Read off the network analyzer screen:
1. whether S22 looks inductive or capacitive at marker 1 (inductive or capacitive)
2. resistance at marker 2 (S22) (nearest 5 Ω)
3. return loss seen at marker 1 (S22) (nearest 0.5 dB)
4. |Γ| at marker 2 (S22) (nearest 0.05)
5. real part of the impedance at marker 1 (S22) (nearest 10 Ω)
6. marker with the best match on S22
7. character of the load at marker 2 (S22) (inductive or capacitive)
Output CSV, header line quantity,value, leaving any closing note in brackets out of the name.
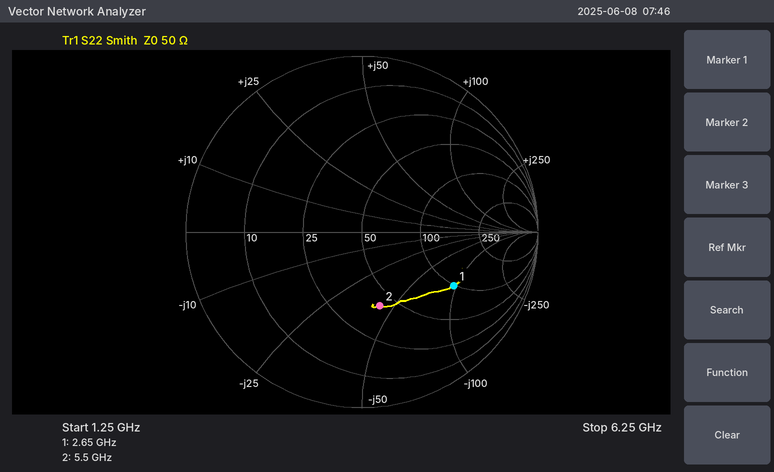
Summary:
quantity,value
whether S22 looks inductive or capacitive at marker 1,capacitive
resistance at marker 2 (S22),40 Ω
return loss seen at marker 1 (S22),4.5 dB
|Γ| at marker 2 (S22),0.45
real part of the impedance at marker 1 (S22),100 Ω
marker with the best match on S22,marker 2
character of the load at marker 2 (S22),capacitive
